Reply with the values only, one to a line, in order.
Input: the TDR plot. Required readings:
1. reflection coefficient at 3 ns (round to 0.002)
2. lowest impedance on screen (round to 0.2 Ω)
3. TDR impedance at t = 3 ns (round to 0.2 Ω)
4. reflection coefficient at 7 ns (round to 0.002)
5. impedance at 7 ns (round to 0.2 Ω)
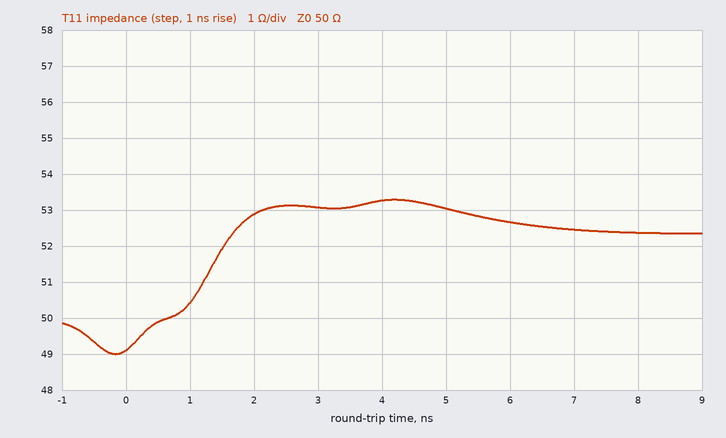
+0.030
49.0 Ω
53.0 Ω
+0.024
52.4 Ω
